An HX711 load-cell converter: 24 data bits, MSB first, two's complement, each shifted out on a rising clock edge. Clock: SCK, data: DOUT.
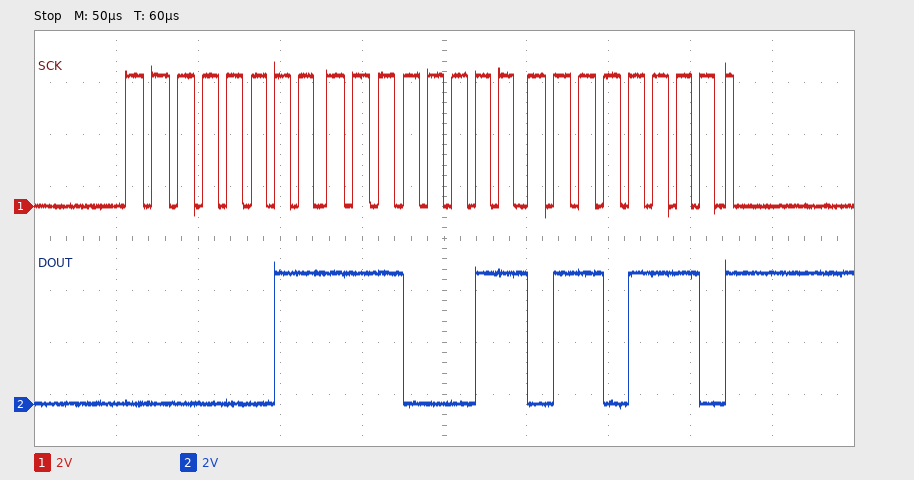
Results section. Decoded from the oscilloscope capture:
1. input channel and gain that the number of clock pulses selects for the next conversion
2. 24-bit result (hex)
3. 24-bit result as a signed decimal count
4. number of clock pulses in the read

channel A, gain 128
0x03E36E
254830
25
